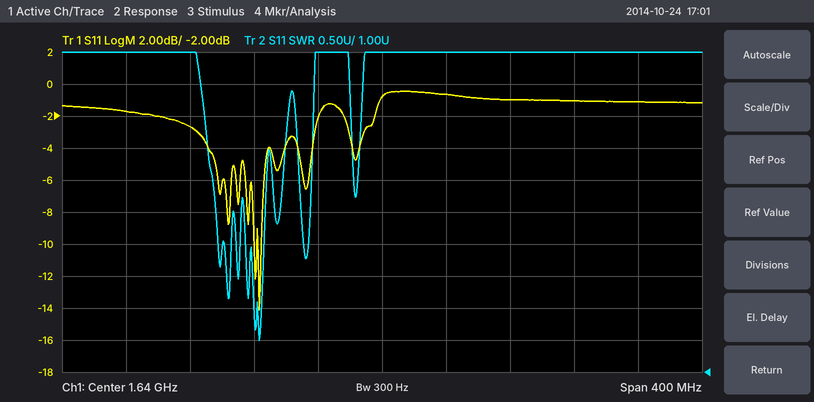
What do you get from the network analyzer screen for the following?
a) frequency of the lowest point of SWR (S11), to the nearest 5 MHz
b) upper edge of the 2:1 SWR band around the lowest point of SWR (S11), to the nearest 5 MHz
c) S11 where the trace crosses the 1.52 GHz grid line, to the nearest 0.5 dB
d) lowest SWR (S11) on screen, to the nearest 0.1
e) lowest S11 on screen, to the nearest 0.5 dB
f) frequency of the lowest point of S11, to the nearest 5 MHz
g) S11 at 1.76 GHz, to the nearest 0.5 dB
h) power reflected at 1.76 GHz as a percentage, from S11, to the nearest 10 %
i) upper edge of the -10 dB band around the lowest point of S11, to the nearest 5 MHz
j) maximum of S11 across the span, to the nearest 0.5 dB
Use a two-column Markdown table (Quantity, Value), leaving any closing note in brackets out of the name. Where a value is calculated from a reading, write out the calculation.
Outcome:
| Quantity | Value |
|---|---|
| frequency of the lowest point of SWR (S11), to the nearest 5 MHz | 1.565 GHz |
| upper edge of the 2:1 SWR band around the lowest point of SWR (S11), to the nearest 5 MHz | 1.565 GHz |
| S11 where the trace crosses the 1.52 GHz grid line, to the nearest 0.5 dB | -2.5 dB |
| lowest SWR (S11) on screen, to the nearest 0.1 | 1.5 |
| lowest S11 on screen, to the nearest 0.5 dB | -14.0 dB |
| frequency of the lowest point of S11, to the nearest 5 MHz | 1.565 GHz |
| S11 at 1.76 GHz, to the nearest 0.5 dB | -1.0 dB |
| power reflected at 1.76 GHz as a percentage, from S11, to the nearest 10 % | 10^(-1/10) ≈ 79.4 %, so 80 % to the nearest 10 % |
| upper edge of the -10 dB band around the lowest point of S11, to the nearest 5 MHz | 1.565 GHz |
| maximum of S11 across the span, to the nearest 0.5 dB | -0.5 dB |
